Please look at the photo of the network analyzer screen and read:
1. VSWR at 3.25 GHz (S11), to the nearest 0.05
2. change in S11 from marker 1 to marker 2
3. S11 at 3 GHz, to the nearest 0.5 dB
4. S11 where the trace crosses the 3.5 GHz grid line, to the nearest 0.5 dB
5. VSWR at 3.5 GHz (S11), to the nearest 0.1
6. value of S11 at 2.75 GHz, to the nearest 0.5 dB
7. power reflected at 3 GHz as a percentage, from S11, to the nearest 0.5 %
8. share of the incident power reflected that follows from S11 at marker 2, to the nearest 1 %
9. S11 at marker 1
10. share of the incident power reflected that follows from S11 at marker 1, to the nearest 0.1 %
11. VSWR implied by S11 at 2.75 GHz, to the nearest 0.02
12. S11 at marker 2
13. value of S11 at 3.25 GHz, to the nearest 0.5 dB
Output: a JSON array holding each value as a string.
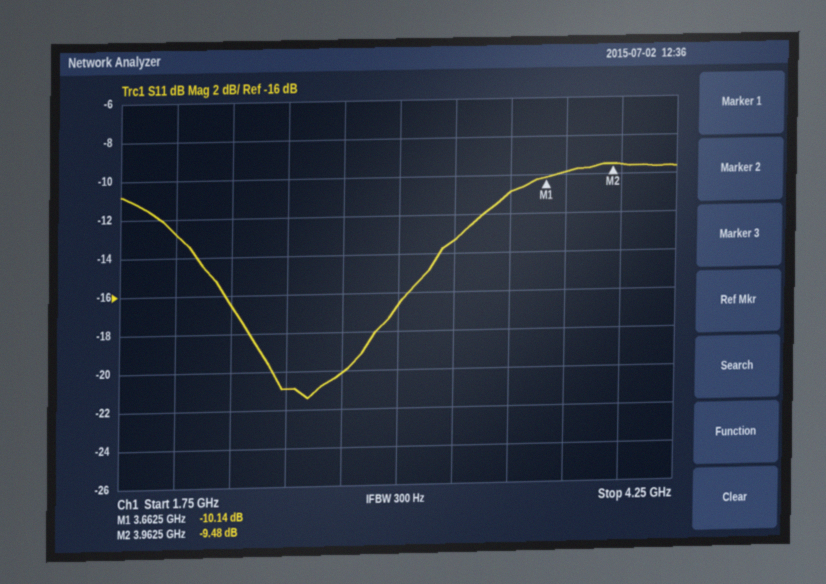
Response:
["1.55", "0.66 dB", "-16.5 dB", "-11.0 dB", "1.8", "-20.0 dB", "2.0 %", "11 %", "-10.14 dB", "9.7 %", "1.22", "-9.48 dB", "-13.5 dB"]
